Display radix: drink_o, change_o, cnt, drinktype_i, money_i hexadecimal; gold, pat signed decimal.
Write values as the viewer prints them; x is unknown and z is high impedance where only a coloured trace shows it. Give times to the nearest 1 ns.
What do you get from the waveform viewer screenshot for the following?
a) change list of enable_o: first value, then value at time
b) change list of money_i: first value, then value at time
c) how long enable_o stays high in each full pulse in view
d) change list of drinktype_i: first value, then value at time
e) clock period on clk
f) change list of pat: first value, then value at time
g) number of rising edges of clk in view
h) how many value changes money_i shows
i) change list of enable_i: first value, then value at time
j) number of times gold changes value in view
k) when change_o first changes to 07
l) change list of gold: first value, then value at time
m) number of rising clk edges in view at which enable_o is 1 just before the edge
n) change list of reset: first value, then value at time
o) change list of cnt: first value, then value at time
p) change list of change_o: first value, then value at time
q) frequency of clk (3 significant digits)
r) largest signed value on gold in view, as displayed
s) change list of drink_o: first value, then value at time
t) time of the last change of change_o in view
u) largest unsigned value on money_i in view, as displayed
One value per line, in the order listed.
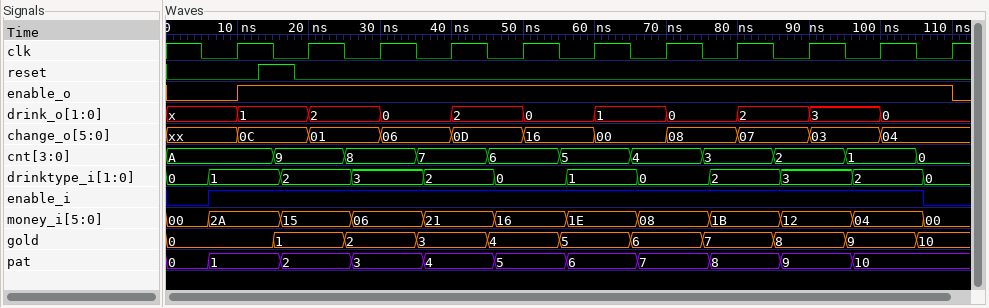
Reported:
0, 1 at 10 ns, 0 at 110 ns
00, 2A at 6 ns, 15 at 16 ns, 06 at 26 ns, 21 at 36 ns, 16 at 46 ns, 1E at 56 ns, 08 at 66 ns, 1B at 76 ns, 12 at 86 ns, 04 at 96 ns, 00 at 106 ns
100 ns
0, 1 at 6 ns, 2 at 16 ns, 3 at 26 ns, 2 at 36 ns, 0 at 46 ns, 1 at 56 ns, 0 at 66 ns, 2 at 76 ns, 3 at 86 ns, 2 at 96 ns, 0 at 106 ns
10 ns
0, 1 at 6 ns, 2 at 16 ns, 3 at 26 ns, 4 at 36 ns, 5 at 46 ns, 6 at 56 ns, 7 at 66 ns, 8 at 76 ns, 9 at 86 ns, 10 at 96 ns
11
11
0, 1 at 6 ns, 0 at 106 ns
10
80 ns
0, 1 at 15 ns, 2 at 25 ns, 3 at 35 ns, 4 at 45 ns, 5 at 55 ns, 6 at 65 ns, 7 at 75 ns, 8 at 85 ns, 9 at 95 ns, 10 at 105 ns
10
0, 1 at 13 ns, 0 at 18 ns
A, 9 at 15 ns, 8 at 25 ns, 7 at 35 ns, 6 at 45 ns, 5 at 55 ns, 4 at 65 ns, 3 at 75 ns, 2 at 85 ns, 1 at 95 ns, 0 at 105 ns
xx, 0C at 10 ns, 01 at 20 ns, 06 at 30 ns, 0D at 40 ns, 16 at 50 ns, 00 at 60 ns, 08 at 70 ns, 07 at 80 ns, 03 at 90 ns, 04 at 100 ns
100 MHz
10
x, 1 at 10 ns, 2 at 20 ns, 0 at 30 ns, 2 at 40 ns, 0 at 50 ns, 1 at 60 ns, 0 at 70 ns, 2 at 80 ns, 3 at 90 ns, 0 at 100 ns
100 ns
2A
